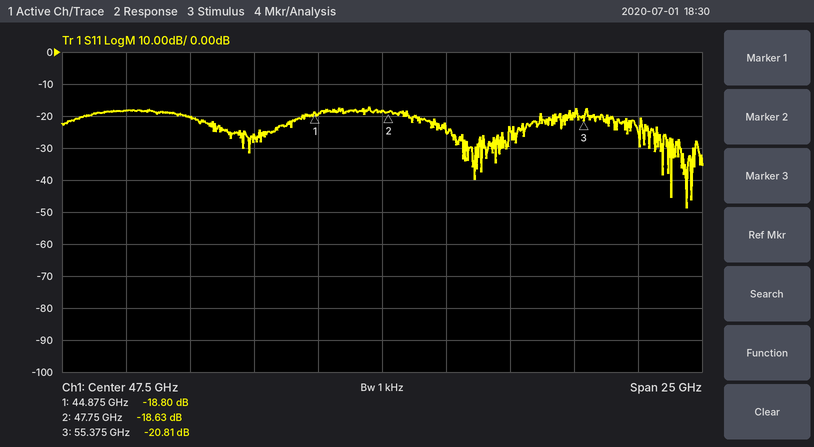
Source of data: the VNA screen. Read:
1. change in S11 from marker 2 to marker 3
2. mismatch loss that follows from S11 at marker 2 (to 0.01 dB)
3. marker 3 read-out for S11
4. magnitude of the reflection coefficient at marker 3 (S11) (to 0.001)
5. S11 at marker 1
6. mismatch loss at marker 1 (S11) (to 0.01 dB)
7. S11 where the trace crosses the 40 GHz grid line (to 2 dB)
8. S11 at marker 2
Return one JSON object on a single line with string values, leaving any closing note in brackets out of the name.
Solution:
{"change in S11 from marker 2 to marker 3": "-2.18 dB", "mismatch loss that follows from S11 at marker 2": "0.06 dB", "marker 3 read-out for S11": "-20.81 dB", "magnitude of the reflection coefficient at marker 3 (S11)": "0.091", "S11 at marker 1": "-18.80 dB", "mismatch loss at marker 1 (S11)": "0.06 dB", "S11 where the trace crosses the 40 GHz grid line": "-20 dB", "S11 at marker 2": "-18.63 dB"}
